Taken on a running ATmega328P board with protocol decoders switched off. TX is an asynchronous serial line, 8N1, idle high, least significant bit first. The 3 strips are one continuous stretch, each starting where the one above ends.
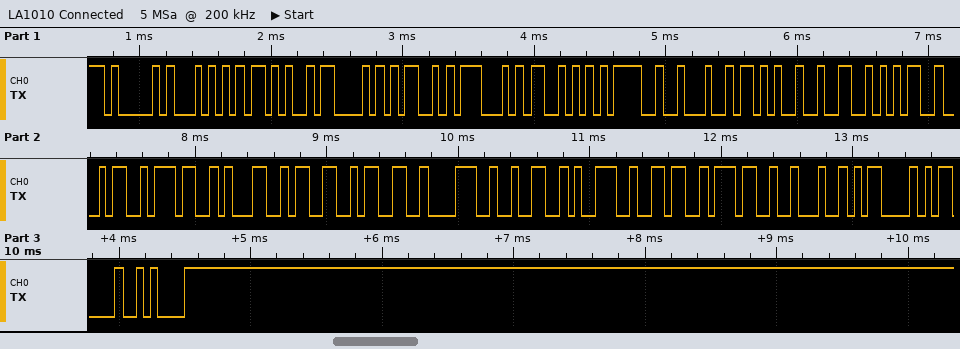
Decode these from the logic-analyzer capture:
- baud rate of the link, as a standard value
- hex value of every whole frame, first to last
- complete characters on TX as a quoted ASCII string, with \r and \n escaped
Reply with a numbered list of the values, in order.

1. 19200 baud
2. 0x41 0x54 0x2B 0x43 0x4D 0x47 0x53 0x3D 0x22 0x2B 0x32 0x35 0x34 0x37 0x31 0x33 0x33 0x38 0x32 0x39 0x36 0x37 0x22 0x0D 0x0D 0x0A
3. "AT+CMGS=\"+254713382967\"\r\r\n"
